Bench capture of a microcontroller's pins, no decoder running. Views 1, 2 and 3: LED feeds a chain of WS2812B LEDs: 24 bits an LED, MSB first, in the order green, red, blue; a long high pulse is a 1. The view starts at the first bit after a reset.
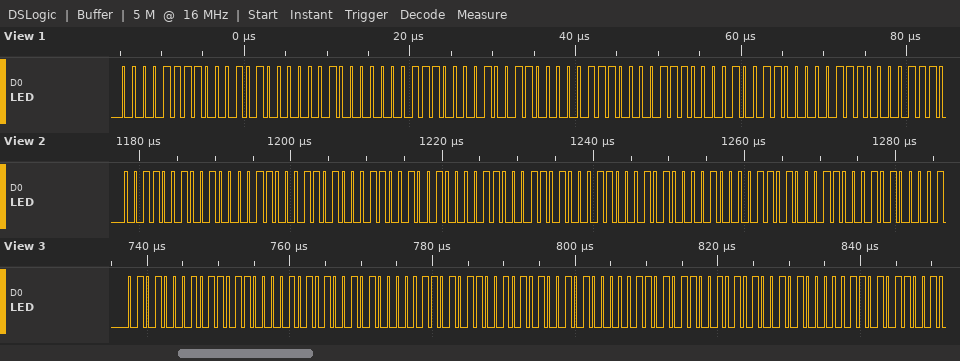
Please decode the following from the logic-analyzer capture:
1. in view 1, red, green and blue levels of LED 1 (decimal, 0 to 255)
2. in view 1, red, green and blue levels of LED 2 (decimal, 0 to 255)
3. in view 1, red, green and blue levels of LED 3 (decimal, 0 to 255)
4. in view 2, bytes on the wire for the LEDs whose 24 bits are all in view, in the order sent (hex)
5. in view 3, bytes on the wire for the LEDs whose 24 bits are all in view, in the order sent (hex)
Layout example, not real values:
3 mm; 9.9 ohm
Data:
20, 15, 8; 19, 14, 7; 19, 14, 7; 32 43 1A 32 43 1A 31 42 1A; 51 6C 2A 50 6B 2A 50 6B 2A
